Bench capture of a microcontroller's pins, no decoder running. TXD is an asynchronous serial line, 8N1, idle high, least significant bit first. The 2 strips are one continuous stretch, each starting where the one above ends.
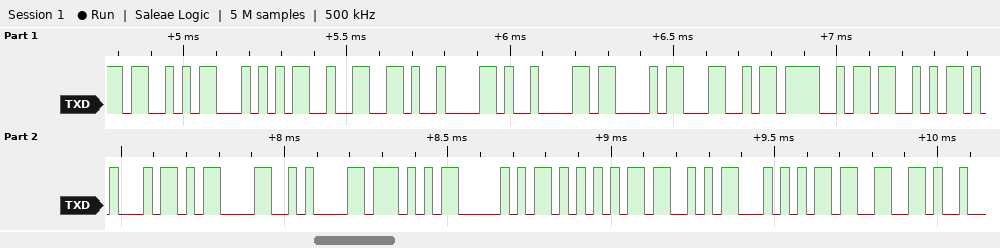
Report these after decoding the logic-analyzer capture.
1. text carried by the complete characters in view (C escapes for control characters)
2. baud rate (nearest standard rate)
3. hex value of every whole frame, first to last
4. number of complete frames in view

"ST2\t\tCLOSE\r\nWPUST3"
38400 baud
53 54 32 09 09 43 4C 4F 53 45 0D 0A 57 50 55 53 54 33
18
